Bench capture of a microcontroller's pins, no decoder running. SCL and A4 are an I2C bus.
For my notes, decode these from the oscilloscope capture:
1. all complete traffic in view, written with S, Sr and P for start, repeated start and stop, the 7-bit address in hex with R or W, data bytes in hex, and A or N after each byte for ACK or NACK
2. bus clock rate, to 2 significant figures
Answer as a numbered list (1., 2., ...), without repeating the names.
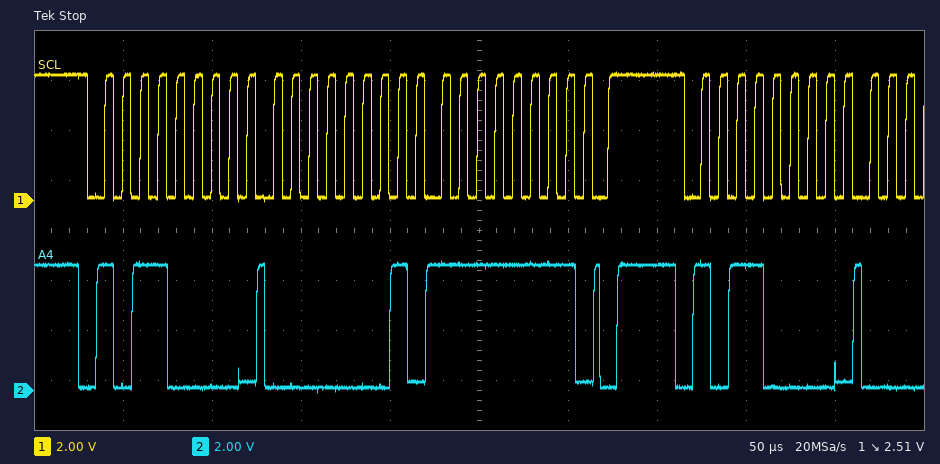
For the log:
1. S 58W A 01 A FF A P S 58W A
2. 100 kHz
